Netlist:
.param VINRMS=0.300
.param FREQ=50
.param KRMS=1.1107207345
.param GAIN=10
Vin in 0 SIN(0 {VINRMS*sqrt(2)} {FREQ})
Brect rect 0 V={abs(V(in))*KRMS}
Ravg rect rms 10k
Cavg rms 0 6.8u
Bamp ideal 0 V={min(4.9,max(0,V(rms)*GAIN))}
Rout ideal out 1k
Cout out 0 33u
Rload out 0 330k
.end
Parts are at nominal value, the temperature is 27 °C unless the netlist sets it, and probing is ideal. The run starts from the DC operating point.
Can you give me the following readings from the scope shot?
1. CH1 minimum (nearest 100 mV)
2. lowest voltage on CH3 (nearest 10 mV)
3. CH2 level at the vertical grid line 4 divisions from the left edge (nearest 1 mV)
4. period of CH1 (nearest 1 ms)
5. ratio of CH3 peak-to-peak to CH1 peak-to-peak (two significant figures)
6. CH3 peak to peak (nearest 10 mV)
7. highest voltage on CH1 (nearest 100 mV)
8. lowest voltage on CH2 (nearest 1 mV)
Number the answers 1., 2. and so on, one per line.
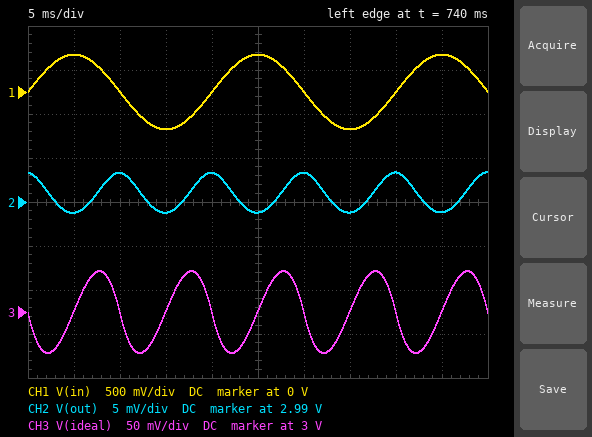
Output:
1. -400 mV
2. 2.95 V
3. 2.993 V
4. 20 ms
5. 0.11
6. 90 mV
7. 400 mV
8. 2.989 V
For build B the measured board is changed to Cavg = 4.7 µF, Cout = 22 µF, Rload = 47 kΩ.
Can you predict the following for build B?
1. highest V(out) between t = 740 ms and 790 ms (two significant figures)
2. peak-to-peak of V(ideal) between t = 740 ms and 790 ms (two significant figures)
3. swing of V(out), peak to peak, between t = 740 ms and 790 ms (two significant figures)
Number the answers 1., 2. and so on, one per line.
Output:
1. 2.9 V
2. 130 mV
3. 9.9 mV
